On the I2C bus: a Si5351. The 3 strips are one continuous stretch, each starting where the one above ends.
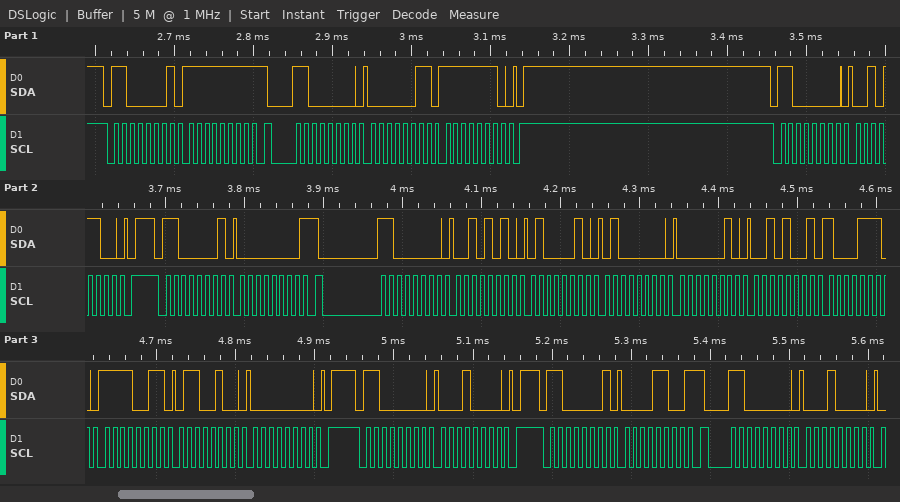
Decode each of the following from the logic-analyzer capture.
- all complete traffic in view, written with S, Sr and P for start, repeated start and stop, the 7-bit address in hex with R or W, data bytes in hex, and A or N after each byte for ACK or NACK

S 60R A FF N Sr 60W A 03 A FE A P S 60W A 2C A P S 60R A 00 N Sr 60W A 2A A 42 A 40 A 02 A 29 A 8E A F3 A 64 A 00 A P S 60W A 10 A P S 60R A 0C N Sr 60W A 10 A
